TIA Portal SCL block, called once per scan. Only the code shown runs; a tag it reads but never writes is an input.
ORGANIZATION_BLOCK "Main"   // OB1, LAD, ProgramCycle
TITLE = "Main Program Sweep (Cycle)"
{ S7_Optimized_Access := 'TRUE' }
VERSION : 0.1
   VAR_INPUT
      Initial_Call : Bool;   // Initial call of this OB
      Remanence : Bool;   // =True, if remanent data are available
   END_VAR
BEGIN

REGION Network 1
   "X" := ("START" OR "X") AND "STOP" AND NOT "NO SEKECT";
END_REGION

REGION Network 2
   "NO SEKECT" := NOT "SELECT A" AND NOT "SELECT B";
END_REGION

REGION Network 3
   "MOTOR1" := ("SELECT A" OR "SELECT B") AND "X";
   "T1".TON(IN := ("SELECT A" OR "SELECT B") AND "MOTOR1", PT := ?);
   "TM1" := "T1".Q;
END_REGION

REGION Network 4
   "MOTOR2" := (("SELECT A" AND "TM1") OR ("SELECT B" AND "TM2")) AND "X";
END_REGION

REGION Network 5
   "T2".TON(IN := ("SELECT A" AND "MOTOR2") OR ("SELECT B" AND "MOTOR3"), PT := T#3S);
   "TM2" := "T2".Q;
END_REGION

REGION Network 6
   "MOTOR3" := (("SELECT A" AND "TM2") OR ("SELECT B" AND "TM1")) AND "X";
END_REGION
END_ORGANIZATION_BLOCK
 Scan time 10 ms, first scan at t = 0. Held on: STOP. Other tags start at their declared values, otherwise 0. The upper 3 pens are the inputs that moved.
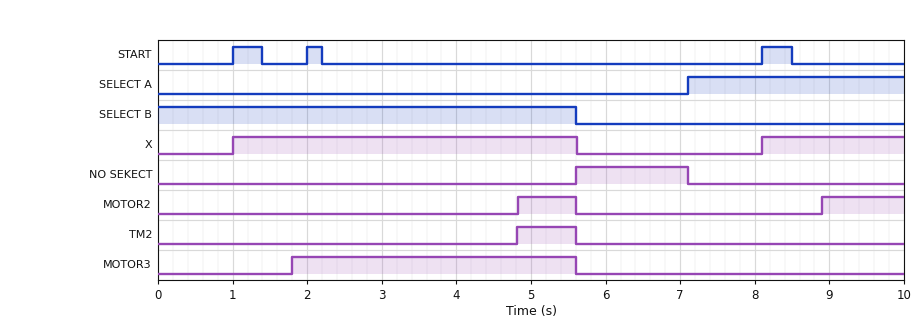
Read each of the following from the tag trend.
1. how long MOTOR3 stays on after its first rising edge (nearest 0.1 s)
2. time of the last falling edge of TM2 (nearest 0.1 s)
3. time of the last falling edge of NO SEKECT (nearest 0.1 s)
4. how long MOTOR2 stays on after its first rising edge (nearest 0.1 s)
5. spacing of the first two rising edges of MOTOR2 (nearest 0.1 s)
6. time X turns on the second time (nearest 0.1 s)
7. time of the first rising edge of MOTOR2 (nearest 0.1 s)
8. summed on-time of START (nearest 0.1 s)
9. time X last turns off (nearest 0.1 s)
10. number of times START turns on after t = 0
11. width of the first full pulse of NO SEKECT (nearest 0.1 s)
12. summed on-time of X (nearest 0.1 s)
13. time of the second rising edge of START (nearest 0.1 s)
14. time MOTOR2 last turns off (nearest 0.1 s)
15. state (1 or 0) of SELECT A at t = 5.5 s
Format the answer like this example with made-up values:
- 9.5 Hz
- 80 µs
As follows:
- 3.8 s
- 5.6 s
- 7.1 s
- 0.8 s
- 4.1 s
- 8.1 s
- 4.8 s
- 1.0 s
- 5.6 s
- 3
- 1.5 s
- 6.5 s
- 2.0 s
- 5.6 s
- 0
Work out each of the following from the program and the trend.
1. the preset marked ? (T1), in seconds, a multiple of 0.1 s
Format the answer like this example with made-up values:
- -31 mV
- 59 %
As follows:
- 0.8 s
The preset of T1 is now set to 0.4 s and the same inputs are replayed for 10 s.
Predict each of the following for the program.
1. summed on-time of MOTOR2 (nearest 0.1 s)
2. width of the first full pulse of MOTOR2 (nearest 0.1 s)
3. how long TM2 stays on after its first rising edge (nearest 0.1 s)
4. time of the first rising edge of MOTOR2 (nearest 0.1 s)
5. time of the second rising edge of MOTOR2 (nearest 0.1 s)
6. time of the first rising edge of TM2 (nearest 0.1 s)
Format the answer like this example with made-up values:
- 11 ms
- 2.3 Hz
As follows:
- 2.7 s
- 1.2 s
- 1.2 s
- 4.4 s
- 8.5 s
- 4.4 s
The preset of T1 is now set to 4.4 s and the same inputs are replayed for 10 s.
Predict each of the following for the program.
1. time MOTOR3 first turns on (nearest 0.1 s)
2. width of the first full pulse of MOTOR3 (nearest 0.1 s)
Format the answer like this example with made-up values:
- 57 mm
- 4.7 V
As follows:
- 5.4 s
- 0.2 s
